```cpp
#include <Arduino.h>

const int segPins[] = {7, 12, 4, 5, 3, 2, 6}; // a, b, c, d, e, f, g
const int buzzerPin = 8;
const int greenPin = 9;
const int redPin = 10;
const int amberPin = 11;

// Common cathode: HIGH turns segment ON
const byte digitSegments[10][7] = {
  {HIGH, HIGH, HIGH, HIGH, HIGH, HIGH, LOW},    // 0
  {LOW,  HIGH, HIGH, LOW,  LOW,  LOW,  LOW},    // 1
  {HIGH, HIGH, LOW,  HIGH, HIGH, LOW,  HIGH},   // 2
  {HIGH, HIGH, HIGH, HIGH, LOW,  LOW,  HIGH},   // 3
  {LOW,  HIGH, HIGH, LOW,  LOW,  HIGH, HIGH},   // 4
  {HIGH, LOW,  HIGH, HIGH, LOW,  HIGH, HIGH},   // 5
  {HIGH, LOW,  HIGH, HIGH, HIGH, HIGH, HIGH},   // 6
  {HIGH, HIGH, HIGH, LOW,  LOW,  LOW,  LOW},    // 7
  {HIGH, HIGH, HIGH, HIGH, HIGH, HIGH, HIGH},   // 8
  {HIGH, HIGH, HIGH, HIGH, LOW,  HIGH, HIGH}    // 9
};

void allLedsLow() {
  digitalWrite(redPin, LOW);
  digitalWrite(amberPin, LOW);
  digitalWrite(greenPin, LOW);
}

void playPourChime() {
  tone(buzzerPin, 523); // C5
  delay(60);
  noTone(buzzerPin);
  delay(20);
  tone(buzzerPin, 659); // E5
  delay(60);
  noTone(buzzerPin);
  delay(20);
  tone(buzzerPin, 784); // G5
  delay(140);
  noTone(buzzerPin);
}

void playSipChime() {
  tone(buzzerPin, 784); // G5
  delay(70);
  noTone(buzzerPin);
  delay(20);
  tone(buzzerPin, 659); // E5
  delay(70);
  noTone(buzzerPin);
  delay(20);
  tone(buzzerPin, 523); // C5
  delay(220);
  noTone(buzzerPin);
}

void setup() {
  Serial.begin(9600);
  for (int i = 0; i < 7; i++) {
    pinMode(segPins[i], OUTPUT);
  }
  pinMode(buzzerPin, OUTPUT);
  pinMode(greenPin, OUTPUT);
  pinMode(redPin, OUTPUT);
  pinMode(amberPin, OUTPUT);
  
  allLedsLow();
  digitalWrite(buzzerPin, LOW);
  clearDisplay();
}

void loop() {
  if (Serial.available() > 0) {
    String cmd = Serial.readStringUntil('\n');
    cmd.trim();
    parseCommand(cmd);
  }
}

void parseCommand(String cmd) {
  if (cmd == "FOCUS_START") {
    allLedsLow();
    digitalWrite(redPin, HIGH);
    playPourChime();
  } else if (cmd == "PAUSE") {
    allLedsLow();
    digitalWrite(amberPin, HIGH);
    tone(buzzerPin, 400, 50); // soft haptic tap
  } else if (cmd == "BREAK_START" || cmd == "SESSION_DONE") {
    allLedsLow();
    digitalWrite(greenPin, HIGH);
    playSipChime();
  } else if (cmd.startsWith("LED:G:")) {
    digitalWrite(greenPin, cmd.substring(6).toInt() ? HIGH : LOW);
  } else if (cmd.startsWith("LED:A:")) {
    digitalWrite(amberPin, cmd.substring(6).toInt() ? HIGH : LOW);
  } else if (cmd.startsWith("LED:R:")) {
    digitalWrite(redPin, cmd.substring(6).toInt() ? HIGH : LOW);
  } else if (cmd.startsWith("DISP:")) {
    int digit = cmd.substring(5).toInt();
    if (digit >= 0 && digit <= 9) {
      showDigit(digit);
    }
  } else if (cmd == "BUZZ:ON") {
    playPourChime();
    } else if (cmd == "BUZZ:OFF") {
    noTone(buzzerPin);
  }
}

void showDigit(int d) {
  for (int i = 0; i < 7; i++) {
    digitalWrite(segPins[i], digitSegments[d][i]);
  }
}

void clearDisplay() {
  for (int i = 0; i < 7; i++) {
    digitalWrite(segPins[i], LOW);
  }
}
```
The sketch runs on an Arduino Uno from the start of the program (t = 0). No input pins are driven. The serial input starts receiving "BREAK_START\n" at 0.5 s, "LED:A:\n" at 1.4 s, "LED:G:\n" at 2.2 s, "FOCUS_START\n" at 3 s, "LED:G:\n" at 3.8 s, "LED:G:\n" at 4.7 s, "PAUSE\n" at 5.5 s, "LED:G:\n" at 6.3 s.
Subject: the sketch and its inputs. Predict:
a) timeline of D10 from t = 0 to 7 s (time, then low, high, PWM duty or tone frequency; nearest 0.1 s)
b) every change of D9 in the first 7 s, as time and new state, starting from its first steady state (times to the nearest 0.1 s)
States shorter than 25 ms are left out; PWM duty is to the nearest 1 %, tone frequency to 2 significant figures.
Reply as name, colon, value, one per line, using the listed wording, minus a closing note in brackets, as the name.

timeline of D10 from t = 0 to 7 s: 0 s low; 3 s high; 5.5 s low
every change of D9 in the first 7 s, as time and new state, starting from its first steady state: 0 s low; 0.5 s high; 2.2 s low
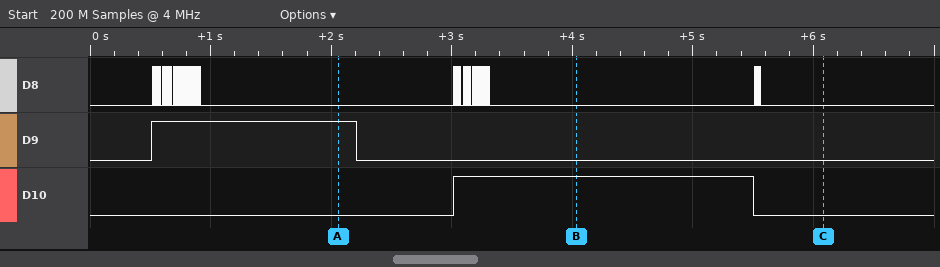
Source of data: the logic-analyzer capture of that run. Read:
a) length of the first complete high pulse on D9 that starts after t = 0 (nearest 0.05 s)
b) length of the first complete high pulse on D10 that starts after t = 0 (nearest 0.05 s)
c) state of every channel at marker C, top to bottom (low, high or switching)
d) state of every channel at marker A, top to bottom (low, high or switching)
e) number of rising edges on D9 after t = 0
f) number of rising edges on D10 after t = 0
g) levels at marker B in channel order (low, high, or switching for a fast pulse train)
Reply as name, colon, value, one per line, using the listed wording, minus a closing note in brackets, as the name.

length of the first complete high pulse on D9 that starts after t = 0: 1.70 s
length of the first complete high pulse on D10 that starts after t = 0: 2.50 s
state of every channel at marker C, top to bottom: D8 low, D9 low, D10 low
state of every channel at marker A, top to bottom: D8 low, D9 high, D10 low
number of rising edges on D9 after t = 0: 1
number of rising edges on D10 after t = 0: 1
levels at marker B in channel order: D8 low, D9 low, D10 high
